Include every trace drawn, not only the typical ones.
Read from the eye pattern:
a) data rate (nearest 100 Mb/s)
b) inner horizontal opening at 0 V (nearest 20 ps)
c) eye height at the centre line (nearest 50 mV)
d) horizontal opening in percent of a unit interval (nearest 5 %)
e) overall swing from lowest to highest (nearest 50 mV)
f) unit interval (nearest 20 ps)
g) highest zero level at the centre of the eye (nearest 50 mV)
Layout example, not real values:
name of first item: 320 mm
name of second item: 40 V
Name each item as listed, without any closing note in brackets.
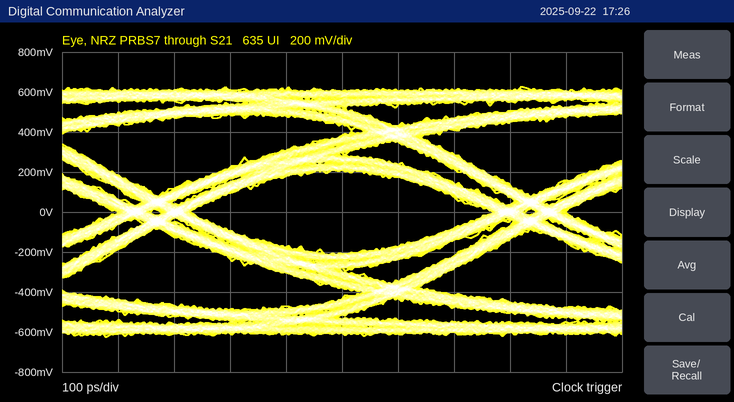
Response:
data rate: 1.5 Gb/s
inner horizontal opening at 0 V: 540 ps
eye height at the centre line: 400 mV
horizontal opening in percent of a unit interval: 80 %
overall swing from lowest to highest: 1.25 V
unit interval: 660 ps
highest zero level at the centre of the eye: -200 mV
